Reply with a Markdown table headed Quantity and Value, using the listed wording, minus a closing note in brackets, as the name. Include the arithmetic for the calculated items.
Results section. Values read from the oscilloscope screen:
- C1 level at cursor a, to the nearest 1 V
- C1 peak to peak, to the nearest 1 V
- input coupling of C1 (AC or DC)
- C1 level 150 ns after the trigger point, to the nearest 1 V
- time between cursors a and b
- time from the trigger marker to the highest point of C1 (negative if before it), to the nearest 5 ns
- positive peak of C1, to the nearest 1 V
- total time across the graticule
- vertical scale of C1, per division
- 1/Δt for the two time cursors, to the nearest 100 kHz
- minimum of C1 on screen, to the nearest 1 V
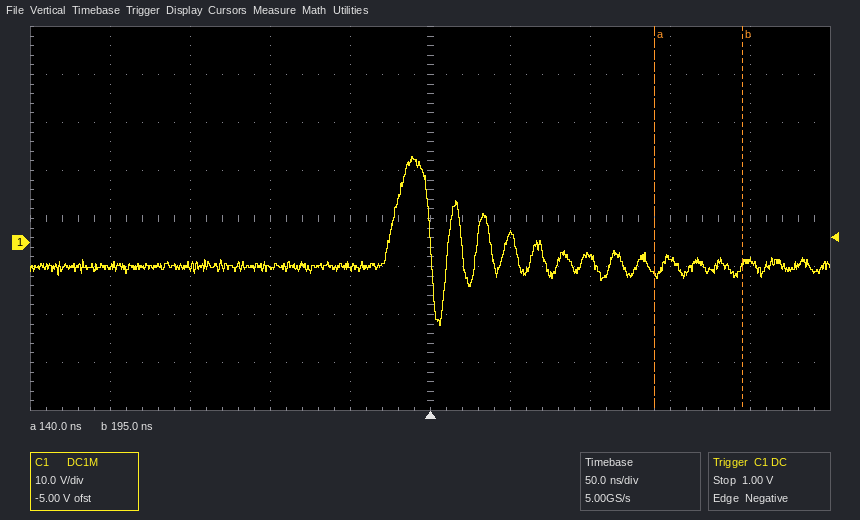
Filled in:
| Quantity | Value |
|---|---|
| C1 level at cursor a, to the nearest 1 V | -7 V |
| C1 peak to peak, to the nearest 1 V | 18 V − (-17 V) = 35 V |
| input coupling of C1 | DC |
| C1 level 150 ns after the trigger point, to the nearest 1 V | -3 V |
| time between cursors a and b | 195 ns − (140 ns) = 55 ns |
| time from the trigger marker to the highest point of C1 (negative if before it), to the nearest 5 ns | -10 ns |
| positive peak of C1, to the nearest 1 V | 18 V |
| total time across the graticule | 500 ns |
| vertical scale of C1, per division | 10 V |
| 1/Δt for the two time cursors, to the nearest 100 kHz | 1 / 55 ns ≈ 18.2 MHz |
| minimum of C1 on screen, to the nearest 1 V | -17 V |
